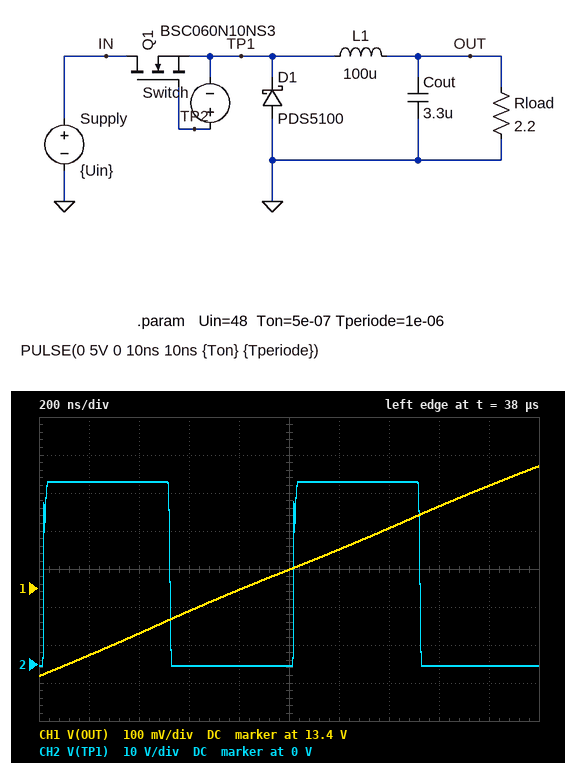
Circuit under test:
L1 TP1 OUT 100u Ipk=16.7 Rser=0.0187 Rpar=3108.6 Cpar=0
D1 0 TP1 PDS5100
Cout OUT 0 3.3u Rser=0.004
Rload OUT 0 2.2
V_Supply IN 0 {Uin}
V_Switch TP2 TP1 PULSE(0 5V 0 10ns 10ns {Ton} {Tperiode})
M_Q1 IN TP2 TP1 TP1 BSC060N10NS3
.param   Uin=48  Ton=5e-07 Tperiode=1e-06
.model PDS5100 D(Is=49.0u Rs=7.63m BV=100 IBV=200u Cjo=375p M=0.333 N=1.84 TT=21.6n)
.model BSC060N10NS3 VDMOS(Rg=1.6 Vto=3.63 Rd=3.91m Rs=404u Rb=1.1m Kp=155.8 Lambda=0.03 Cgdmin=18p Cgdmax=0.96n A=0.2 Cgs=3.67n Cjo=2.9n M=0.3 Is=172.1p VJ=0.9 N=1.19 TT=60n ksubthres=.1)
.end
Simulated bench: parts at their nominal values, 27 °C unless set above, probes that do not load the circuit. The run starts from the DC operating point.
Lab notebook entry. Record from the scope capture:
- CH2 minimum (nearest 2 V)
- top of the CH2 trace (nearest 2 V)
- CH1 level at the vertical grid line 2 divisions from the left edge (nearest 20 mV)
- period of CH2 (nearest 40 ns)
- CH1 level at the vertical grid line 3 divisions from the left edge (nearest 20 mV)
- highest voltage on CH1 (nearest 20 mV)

0 V
48 V
13.28 V
1.00 µs
13.34 V
13.72 V
